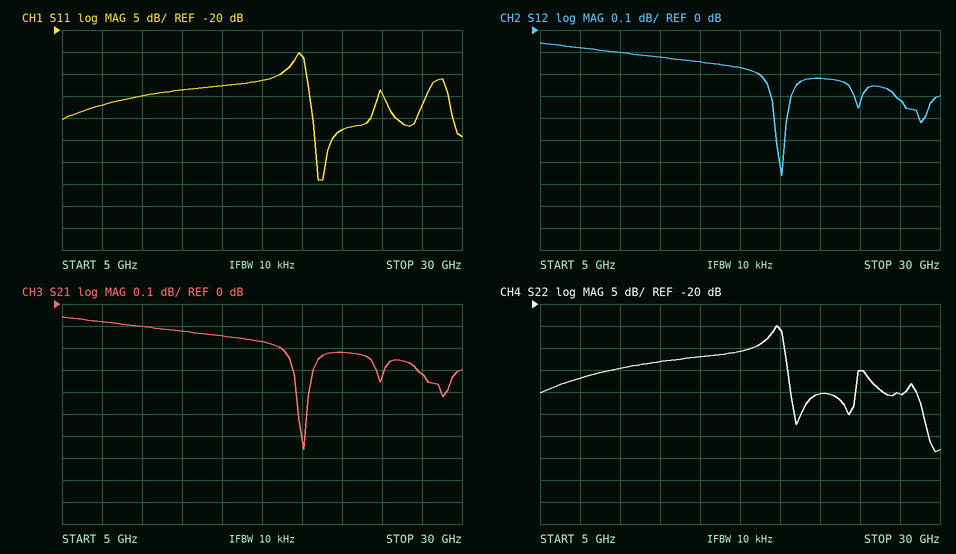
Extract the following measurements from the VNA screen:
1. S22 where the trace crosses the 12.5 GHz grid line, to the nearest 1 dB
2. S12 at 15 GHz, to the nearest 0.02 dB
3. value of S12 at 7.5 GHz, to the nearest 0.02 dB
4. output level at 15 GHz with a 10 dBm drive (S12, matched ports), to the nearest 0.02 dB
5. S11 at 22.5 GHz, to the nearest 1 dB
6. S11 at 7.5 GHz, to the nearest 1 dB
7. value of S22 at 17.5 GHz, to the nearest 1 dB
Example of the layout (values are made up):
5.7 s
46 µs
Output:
-33 dB
-0.14 dB
-0.08 dB
9.86 dBm
-43 dB
-37 dB
-31 dB
